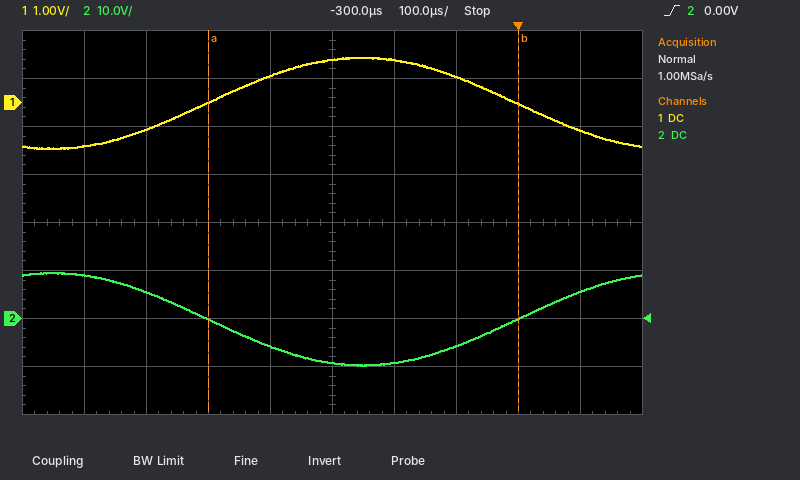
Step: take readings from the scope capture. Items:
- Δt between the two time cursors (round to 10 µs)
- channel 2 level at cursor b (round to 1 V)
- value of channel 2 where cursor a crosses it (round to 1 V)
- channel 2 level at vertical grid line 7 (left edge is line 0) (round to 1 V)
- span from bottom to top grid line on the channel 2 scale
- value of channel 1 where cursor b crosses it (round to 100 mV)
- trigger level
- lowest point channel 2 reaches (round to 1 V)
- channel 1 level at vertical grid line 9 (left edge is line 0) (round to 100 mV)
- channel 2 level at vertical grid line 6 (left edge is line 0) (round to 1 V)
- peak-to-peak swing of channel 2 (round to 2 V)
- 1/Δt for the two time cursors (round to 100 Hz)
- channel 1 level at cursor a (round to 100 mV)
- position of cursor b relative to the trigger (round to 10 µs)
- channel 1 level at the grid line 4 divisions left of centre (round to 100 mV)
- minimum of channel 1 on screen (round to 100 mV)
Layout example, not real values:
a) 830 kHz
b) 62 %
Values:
a) 500 µs
b) 0 V
c) 0 V
d) -6 V
e) 80 V
f) 0.0 V
g) 0.00 V
h) -10 V
i) -600 mV
j) -9 V
k) 20 V
l) 2.0 kHz
m) 0.0 V
n) 0 µs
o) -900 mV
p) -1.0 V
